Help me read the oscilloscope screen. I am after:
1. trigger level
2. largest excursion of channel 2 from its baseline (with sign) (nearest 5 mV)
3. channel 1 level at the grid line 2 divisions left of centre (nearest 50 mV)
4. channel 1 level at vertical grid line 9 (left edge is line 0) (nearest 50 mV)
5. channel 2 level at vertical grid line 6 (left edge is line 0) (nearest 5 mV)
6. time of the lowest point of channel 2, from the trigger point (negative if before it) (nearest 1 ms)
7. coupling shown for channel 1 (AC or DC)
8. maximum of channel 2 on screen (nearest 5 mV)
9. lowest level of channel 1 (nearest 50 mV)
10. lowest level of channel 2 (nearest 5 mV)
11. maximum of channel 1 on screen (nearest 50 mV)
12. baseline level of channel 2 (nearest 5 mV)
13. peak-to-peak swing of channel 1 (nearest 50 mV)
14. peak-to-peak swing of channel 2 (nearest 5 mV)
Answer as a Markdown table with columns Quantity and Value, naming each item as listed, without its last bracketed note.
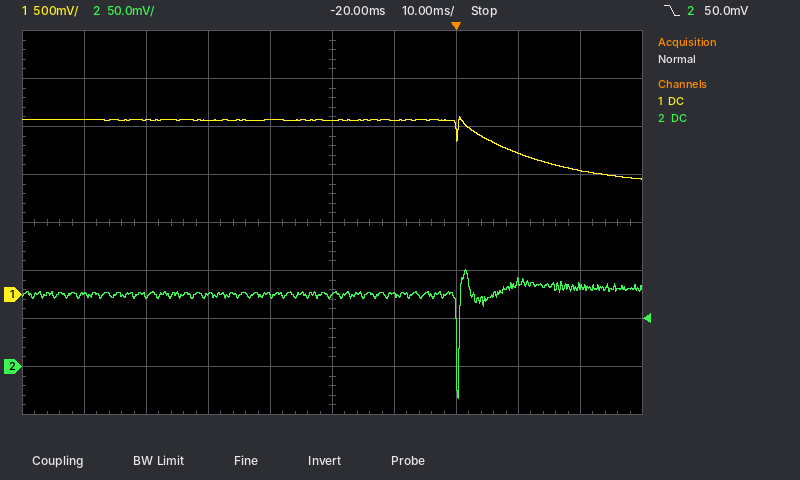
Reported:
| Quantity | Value |
|---|---|
| trigger level | 50.0 mV |
| largest excursion of channel 2 from its baseline (with sign) | -110 mV |
| channel 1 level at the grid line 2 divisions left of centre | 1.80 V |
| channel 1 level at vertical grid line 9 (left edge is line 0) | 1.30 V |
| channel 2 level at vertical grid line 6 (left edge is line 0) | 75 mV |
| time of the lowest point of channel 2, from the trigger point (negative if before it) | 0 ms |
| coupling shown for channel 1 | DC |
| maximum of channel 2 on screen | 100 mV |
| lowest level of channel 1 | 1.20 V |
| lowest level of channel 2 | -35 mV |
| maximum of channel 1 on screen | 1.85 V |
| baseline level of channel 2 | 75 mV |
| peak-to-peak swing of channel 1 | 650 mV |
| peak-to-peak swing of channel 2 | 135 mV |
